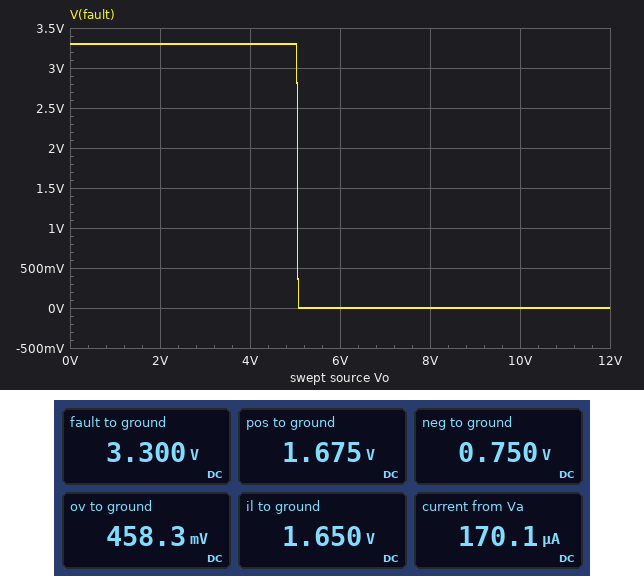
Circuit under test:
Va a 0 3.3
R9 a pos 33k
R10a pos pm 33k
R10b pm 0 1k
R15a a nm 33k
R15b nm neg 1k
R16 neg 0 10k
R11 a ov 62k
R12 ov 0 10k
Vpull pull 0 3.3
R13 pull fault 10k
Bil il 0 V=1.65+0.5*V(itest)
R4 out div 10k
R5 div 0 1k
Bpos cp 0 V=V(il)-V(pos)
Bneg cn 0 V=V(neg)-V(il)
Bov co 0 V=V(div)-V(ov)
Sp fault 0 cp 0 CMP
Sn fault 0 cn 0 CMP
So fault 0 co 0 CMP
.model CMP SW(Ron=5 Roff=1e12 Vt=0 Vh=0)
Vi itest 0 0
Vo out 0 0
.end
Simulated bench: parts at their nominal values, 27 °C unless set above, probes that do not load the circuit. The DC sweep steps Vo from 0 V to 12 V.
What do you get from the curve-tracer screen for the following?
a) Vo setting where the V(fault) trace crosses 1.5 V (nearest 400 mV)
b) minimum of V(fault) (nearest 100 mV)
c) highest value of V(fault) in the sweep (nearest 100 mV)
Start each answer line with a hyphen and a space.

- 5.2 V
- 0 V
- 3.3 V
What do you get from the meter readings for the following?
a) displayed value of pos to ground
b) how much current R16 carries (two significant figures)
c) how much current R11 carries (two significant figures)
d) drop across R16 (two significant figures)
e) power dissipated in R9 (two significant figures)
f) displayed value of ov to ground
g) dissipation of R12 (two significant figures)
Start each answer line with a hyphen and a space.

- 1.675 V
- 75 µA
- 46 µA
- 750 mV
- 80 µW
- 458.3 mV
- 21 µW
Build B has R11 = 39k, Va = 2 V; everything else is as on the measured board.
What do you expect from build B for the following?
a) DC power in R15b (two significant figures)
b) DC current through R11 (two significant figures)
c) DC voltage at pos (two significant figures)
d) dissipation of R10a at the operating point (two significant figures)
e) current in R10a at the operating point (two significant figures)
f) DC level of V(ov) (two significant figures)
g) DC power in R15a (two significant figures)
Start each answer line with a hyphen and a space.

- 2.1 µW
- 41 µA
- 1.0 V
- 29 µW
- 30 µA
- 410 mV
- 68 µW
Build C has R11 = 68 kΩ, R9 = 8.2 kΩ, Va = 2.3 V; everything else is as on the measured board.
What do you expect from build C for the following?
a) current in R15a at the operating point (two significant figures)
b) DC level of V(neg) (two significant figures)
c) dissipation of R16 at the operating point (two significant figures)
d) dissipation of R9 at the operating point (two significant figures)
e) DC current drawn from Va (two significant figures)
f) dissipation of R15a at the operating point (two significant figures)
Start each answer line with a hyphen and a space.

- 52 µA
- 520 mV
- 27 µW
- 24 µW
- 140 µA
- 90 µW
